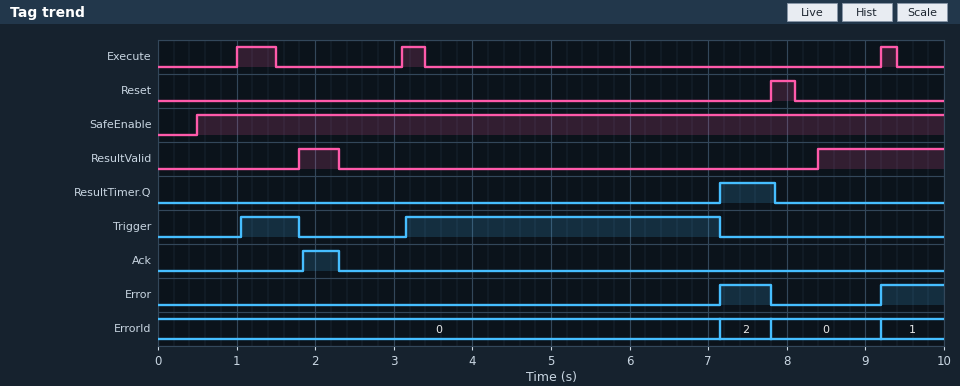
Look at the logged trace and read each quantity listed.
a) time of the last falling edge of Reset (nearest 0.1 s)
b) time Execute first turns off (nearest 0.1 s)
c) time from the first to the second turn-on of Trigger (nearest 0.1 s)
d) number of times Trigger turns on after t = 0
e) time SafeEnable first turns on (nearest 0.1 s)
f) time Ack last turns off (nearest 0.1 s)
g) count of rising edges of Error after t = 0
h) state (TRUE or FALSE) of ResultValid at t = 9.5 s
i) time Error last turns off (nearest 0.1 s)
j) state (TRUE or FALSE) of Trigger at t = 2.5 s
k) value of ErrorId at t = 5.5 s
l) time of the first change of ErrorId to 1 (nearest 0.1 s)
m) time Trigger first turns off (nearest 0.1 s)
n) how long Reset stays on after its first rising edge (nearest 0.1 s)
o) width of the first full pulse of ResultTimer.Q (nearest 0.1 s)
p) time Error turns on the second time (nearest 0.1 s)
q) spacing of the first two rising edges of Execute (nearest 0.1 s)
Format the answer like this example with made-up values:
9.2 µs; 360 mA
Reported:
8.1 s; 1.5 s; 2.1 s; 2; 0.5 s; 2.3 s; 2; TRUE; 7.8 s; FALSE; 0; 9.2 s; 1.8 s; 0.3 s; 0.7 s; 9.2 s; 2.1 s
